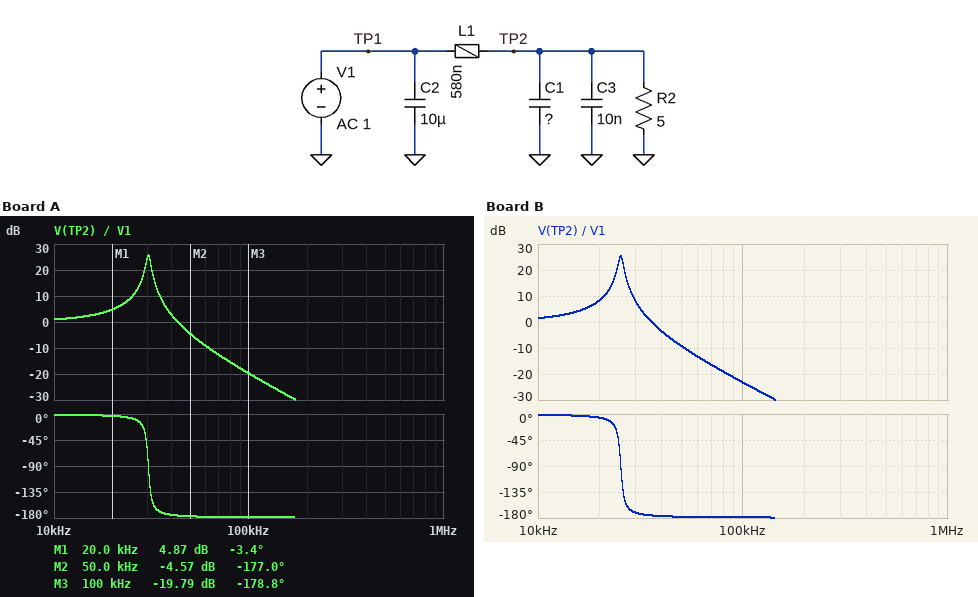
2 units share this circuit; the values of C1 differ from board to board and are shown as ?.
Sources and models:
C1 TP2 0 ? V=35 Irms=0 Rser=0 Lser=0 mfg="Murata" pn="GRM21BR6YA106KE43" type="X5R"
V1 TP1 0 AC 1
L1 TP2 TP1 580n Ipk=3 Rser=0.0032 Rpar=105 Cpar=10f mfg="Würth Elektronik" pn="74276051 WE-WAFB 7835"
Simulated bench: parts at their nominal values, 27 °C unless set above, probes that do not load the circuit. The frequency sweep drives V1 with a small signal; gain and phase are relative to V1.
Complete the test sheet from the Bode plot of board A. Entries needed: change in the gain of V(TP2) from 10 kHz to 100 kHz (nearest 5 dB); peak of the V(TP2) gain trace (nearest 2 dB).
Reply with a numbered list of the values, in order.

1. -20 dB
2. 26 dB
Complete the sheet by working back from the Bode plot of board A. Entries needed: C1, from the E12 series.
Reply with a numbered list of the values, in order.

1. 47 µF
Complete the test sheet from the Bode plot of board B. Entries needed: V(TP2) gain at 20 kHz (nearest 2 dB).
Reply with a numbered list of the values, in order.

1. 8 dB
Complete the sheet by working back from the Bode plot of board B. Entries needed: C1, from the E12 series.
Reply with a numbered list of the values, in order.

1. 68 µF
